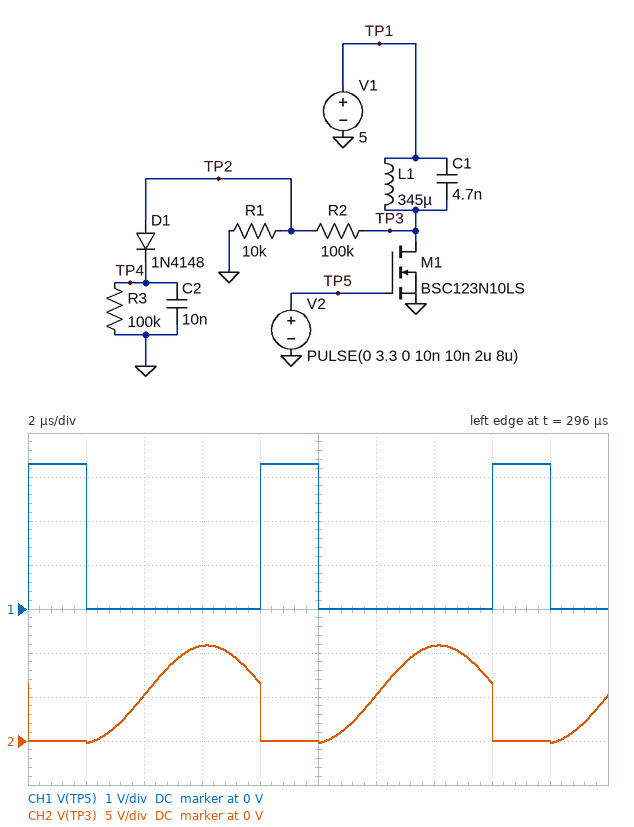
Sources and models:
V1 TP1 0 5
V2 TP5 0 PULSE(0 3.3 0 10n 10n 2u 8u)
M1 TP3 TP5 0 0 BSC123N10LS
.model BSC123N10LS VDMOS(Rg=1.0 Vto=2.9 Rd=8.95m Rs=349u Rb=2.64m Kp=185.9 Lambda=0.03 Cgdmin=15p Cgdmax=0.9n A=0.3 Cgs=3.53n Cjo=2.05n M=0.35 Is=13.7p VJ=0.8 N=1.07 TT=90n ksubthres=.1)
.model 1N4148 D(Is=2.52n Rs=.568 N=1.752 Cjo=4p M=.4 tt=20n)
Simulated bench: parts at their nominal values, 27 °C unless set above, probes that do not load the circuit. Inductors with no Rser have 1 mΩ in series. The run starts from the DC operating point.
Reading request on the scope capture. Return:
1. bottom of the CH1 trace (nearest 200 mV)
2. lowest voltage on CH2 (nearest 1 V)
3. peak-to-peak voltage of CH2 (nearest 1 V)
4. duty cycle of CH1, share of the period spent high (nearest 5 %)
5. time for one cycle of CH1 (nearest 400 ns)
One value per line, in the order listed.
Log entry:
0 V
0 V
11 V
25 %
8.0 µs
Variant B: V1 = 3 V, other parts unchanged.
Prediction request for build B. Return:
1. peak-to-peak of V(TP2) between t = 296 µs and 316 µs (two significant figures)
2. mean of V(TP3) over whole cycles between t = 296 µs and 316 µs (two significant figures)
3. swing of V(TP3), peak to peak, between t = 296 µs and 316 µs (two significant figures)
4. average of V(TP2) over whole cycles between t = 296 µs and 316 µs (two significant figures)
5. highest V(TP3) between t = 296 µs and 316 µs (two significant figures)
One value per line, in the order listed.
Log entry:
520 mV
3.0 V
6.9 V
250 mV
6.6 V
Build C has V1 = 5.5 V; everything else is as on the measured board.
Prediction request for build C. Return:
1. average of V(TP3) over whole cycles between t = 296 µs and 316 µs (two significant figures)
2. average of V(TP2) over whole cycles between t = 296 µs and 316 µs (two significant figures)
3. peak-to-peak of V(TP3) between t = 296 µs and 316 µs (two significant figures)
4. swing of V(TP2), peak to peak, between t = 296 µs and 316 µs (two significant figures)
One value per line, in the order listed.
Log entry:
5.5 V
430 mV
12 V
850 mV
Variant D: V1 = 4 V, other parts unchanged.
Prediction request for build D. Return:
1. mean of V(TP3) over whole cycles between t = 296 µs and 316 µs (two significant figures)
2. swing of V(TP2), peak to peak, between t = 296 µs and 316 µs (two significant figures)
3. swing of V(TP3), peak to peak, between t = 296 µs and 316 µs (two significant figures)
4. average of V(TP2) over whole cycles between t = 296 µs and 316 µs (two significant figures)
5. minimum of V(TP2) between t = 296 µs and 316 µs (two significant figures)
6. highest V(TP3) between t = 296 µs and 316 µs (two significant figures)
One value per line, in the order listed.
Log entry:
4.0 V
650 mV
9.0 V
320 mV
-19 mV
8.7 V
